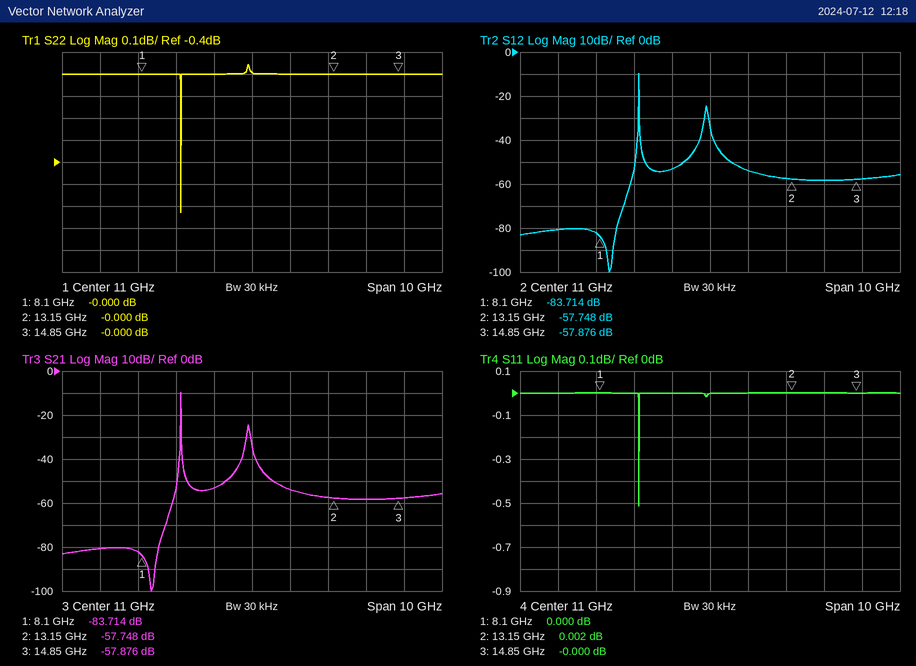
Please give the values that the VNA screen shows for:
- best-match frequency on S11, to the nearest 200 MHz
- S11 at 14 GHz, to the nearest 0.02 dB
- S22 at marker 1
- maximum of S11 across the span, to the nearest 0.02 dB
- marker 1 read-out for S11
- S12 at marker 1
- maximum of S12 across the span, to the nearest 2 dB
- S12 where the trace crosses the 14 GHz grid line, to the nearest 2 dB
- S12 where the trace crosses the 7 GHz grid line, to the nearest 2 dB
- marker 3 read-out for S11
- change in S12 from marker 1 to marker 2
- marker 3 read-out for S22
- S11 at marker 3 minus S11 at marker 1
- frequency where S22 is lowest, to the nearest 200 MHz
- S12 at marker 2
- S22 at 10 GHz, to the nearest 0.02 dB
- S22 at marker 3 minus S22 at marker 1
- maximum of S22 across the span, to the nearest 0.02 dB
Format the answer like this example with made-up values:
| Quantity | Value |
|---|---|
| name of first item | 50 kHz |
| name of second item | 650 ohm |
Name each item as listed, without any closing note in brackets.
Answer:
| Quantity | Value |
|---|---|
| best-match frequency on S11, to the nearest 200 MHz | 9.2 GHz |
| S11 at 14 GHz, to the nearest 0.02 dB | 0.00 dB |
| S22 at marker 1 | -0.000 dB |
| maximum of S11 across the span, to the nearest 0.02 dB | 0.00 dB |
| marker 1 read-out for S11 | 0.000 dB |
| S12 at marker 1 | -83.714 dB |
| maximum of S12 across the span, to the nearest 2 dB | -10 dB |
| S12 where the trace crosses the 14 GHz grid line, to the nearest 2 dB | -58 dB |
| S12 where the trace crosses the 7 GHz grid line, to the nearest 2 dB | -80 dB |
| marker 3 read-out for S11 | -0.000 dB |
| change in S12 from marker 1 to marker 2 | 25.966 dB |
| marker 3 read-out for S22 | -0.000 dB |
| S11 at marker 3 minus S11 at marker 1 | 0.000 dB |
| frequency where S22 is lowest, to the nearest 200 MHz | 9.2 GHz |
| S12 at marker 2 | -57.748 dB |
| S22 at 10 GHz, to the nearest 0.02 dB | 0.00 dB |
| S22 at marker 3 minus S22 at marker 1 | 0.000 dB |
| maximum of S22 across the span, to the nearest 0.02 dB | 0.04 dB |
